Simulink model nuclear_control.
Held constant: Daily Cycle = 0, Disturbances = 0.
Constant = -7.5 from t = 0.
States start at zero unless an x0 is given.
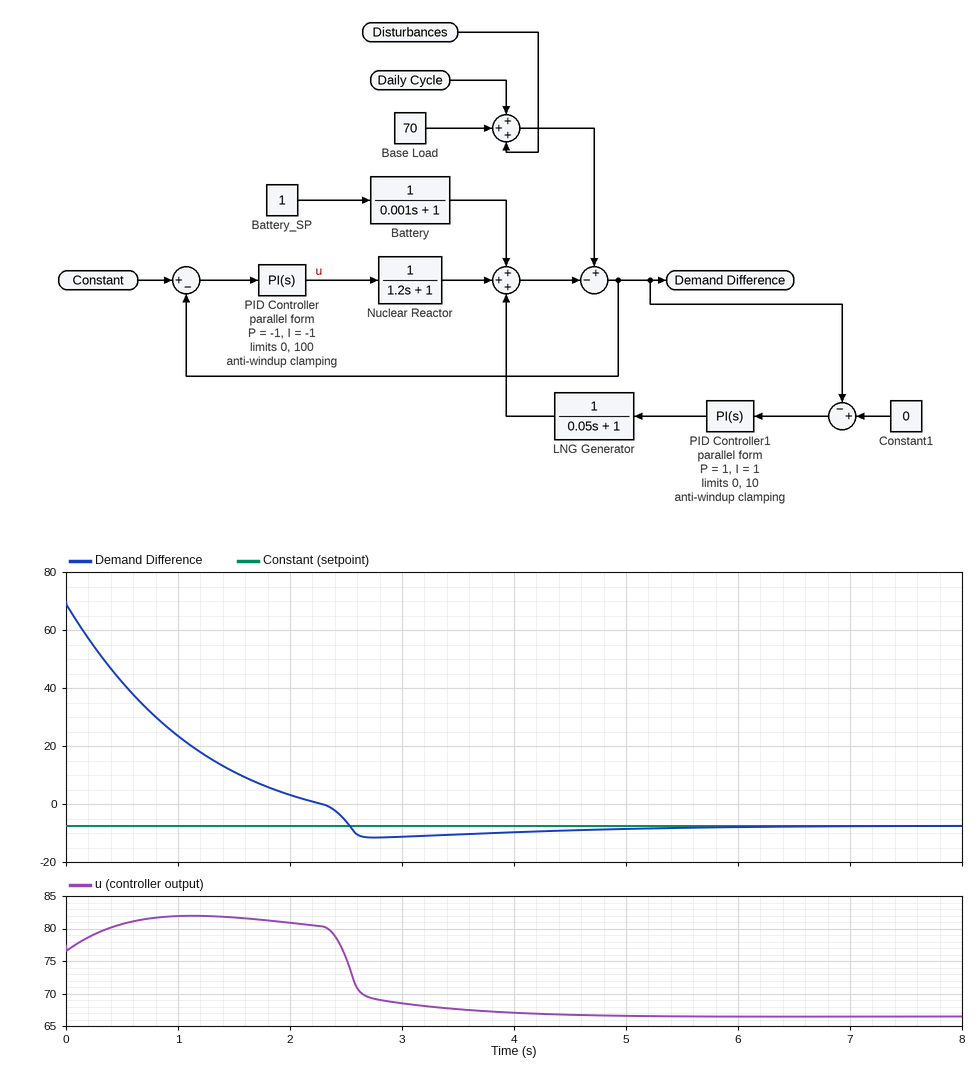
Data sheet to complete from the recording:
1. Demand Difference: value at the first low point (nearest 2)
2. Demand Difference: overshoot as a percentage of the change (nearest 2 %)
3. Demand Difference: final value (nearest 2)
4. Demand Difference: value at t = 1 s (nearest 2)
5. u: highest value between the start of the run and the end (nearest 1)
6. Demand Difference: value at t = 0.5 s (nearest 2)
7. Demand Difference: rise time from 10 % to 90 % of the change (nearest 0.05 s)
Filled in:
-12
6 %
-8
24
82
42
2.15 s
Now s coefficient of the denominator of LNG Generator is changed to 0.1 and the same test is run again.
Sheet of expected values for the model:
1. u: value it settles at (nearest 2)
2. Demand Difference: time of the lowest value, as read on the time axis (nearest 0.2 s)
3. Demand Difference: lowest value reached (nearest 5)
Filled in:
66
3.0 s
-10
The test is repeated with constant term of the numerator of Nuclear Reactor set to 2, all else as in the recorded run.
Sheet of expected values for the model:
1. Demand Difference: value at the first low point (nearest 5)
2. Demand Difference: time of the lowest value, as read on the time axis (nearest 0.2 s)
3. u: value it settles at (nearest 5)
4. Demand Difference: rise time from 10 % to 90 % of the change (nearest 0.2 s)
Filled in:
-10
1.6 s
35
1.2 s
